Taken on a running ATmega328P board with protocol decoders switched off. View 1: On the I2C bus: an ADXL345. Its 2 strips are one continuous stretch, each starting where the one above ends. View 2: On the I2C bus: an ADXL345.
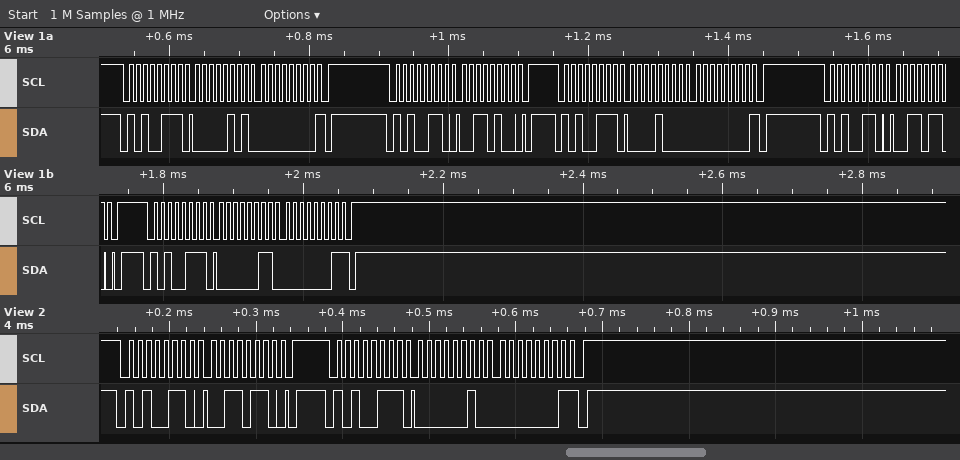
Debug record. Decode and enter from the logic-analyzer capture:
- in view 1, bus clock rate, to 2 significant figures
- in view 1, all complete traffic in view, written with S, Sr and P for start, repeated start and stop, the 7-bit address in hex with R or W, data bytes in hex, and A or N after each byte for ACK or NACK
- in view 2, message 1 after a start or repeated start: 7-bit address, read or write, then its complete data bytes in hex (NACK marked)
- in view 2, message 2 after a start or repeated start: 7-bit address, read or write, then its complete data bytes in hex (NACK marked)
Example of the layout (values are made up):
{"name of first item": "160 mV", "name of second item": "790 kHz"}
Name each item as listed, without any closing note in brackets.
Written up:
{"in view 1, bus clock rate, to 2 significant figures": "100 kHz", "in view 1, all complete traffic in view, written with S, Sr and P for start, repeated start and stop, the 7-bit address in hex with R or W, data bytes in hex, and A or N after each byte for ACK or NACK": "S 53R A 05 A 00 N P S 53W A 34 A P S 53R A 08 A 00 N P S 53W A 36 A P S 53R A 03 A 01 N P", "in view 2, message 1 after a start or repeated start: 7-bit address, read or write, then its complete data bytes in hex": "0x53 write: 36", "in view 2, message 2 after a start or repeated start: 7-bit address, read or write, then its complete data bytes in hex": "0x53 read: 02 01 NACK"}
